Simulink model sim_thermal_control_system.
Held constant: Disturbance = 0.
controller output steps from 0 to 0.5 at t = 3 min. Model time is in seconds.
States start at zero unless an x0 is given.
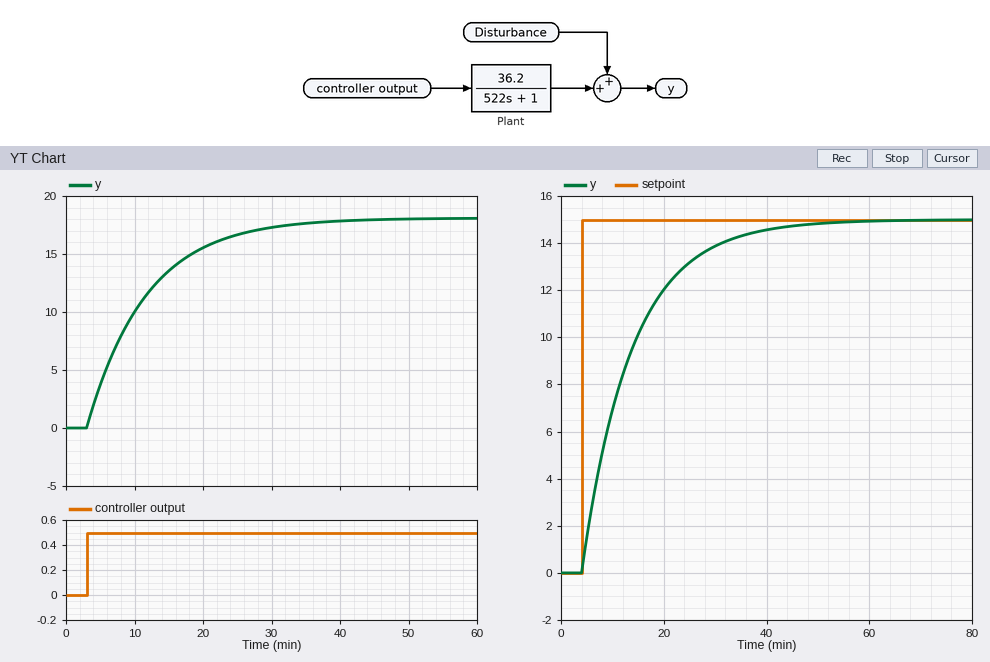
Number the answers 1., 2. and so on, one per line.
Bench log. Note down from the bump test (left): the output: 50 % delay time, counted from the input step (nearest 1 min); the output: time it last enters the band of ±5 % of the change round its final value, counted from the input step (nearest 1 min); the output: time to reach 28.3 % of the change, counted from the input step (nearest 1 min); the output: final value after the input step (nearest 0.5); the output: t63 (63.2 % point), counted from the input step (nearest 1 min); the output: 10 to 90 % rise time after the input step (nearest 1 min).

1. 6 min
2. 26 min
3. 3 min
4. 18.0
5. 9 min
6. 19 min
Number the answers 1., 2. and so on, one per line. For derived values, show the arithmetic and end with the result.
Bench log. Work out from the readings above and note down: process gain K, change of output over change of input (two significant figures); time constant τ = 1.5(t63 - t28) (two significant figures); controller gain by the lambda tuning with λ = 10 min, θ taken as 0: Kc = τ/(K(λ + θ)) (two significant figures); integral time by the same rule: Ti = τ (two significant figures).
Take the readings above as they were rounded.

1. (18 - 0) / 0.5 = 36
2. 1.5 × (9 - 3) = 9.0 min
3. 9 / (36 × (10 + 0)) = 0.025
4. 9.0 min
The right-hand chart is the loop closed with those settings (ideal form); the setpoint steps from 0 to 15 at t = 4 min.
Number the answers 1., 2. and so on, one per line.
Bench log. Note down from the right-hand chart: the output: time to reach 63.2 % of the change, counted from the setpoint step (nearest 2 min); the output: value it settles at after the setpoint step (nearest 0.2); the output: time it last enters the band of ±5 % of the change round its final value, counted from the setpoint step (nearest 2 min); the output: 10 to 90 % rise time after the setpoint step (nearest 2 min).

1. 10 min
2. 15.0
3. 30 min
4. 22 min
